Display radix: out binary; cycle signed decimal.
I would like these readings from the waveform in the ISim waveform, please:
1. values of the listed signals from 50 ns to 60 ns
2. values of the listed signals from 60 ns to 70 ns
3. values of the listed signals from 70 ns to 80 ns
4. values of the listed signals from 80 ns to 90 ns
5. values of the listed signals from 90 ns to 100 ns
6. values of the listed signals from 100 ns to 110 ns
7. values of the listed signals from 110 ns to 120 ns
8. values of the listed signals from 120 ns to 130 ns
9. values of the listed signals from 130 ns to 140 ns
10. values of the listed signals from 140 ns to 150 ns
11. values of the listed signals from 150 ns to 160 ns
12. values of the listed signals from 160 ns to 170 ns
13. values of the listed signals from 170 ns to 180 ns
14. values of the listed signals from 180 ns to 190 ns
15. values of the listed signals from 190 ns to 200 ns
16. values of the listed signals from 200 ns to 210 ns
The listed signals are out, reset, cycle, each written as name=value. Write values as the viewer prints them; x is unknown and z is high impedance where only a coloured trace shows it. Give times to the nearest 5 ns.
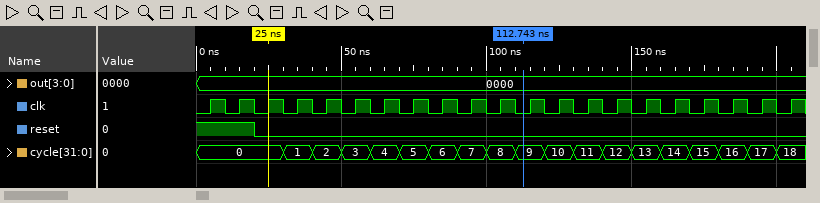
out=0000, reset=0, cycle=3
out=0000, reset=0, cycle=4
out=0000, reset=0, cycle=5
out=0000, reset=0, cycle=6
out=0000, reset=0, cycle=7
out=0000, reset=0, cycle=8
out=0000, reset=0, cycle=9
out=0000, reset=0, cycle=10
out=0000, reset=0, cycle=11
out=0000, reset=0, cycle=12
out=0000, reset=0, cycle=13
out=0000, reset=0, cycle=14
out=0000, reset=0, cycle=15
out=0000, reset=0, cycle=16
out=0000, reset=0, cycle=17
out=0000, reset=0, cycle=18
